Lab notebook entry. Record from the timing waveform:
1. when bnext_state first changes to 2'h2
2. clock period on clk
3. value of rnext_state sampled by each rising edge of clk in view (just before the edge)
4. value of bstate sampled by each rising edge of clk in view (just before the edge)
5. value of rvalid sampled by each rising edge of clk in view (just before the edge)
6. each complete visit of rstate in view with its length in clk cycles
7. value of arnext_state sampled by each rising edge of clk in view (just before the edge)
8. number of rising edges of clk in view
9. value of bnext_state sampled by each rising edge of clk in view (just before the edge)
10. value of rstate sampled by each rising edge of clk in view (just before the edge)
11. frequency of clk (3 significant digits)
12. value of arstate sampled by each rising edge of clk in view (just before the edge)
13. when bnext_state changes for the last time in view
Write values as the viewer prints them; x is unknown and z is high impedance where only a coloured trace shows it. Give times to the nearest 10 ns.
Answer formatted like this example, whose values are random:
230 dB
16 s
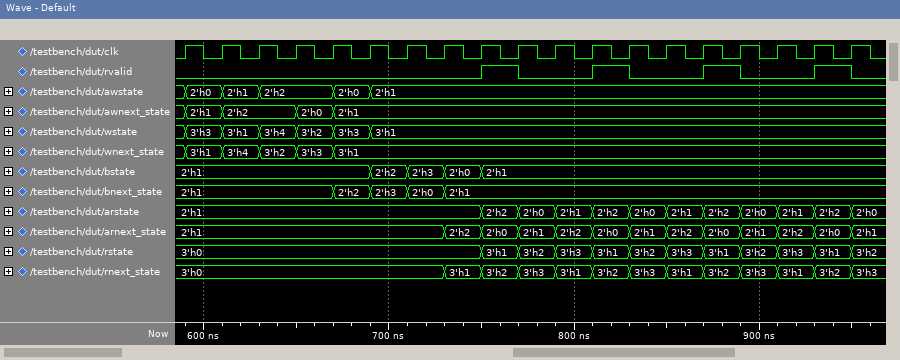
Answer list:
670 ns
20 ns
3'h0, 3'h0, 3'h0, 3'h0, 3'h0, 3'h0, 3'h0, 3'h0, 3'h1, 3'h2, 3'h3, 3'h1, 3'h2, 3'h3, 3'h1, 3'h2, 3'h3, 3'h1, 3'h2
2'h1, 2'h1, 2'h1, 2'h1, 2'h1, 2'h1, 2'h2, 2'h3, 2'h0, 2'h1, 2'h1, 2'h1, 2'h1, 2'h1, 2'h1, 2'h1, 2'h1, 2'h1, 2'h1
0 0 0 0 0 0 0 0 0 1 0 0 1 0 0 1 0 0 1
3'h1: 1, 3'h2: 1, 3'h3: 1, 3'h1: 1, 3'h2: 1, 3'h3: 1, 3'h1: 1, 3'h2: 1, 3'h3: 1, 3'h1: 1
2'h1, 2'h1, 2'h1, 2'h1, 2'h1, 2'h1, 2'h1, 2'h1, 2'h2, 2'h0, 2'h1, 2'h2, 2'h0, 2'h1, 2'h2, 2'h0, 2'h1, 2'h2, 2'h0
19
2'h1, 2'h1, 2'h1, 2'h1, 2'h1, 2'h2, 2'h3, 2'h0, 2'h1, 2'h1, 2'h1, 2'h1, 2'h1, 2'h1, 2'h1, 2'h1, 2'h1, 2'h1, 2'h1
3'h0, 3'h0, 3'h0, 3'h0, 3'h0, 3'h0, 3'h0, 3'h0, 3'h0, 3'h1, 3'h2, 3'h3, 3'h1, 3'h2, 3'h3, 3'h1, 3'h2, 3'h3, 3'h1
50.0 MHz
2'h1, 2'h1, 2'h1, 2'h1, 2'h1, 2'h1, 2'h1, 2'h1, 2'h1, 2'h2, 2'h0, 2'h1, 2'h2, 2'h0, 2'h1, 2'h2, 2'h0, 2'h1, 2'h2
730 ns
